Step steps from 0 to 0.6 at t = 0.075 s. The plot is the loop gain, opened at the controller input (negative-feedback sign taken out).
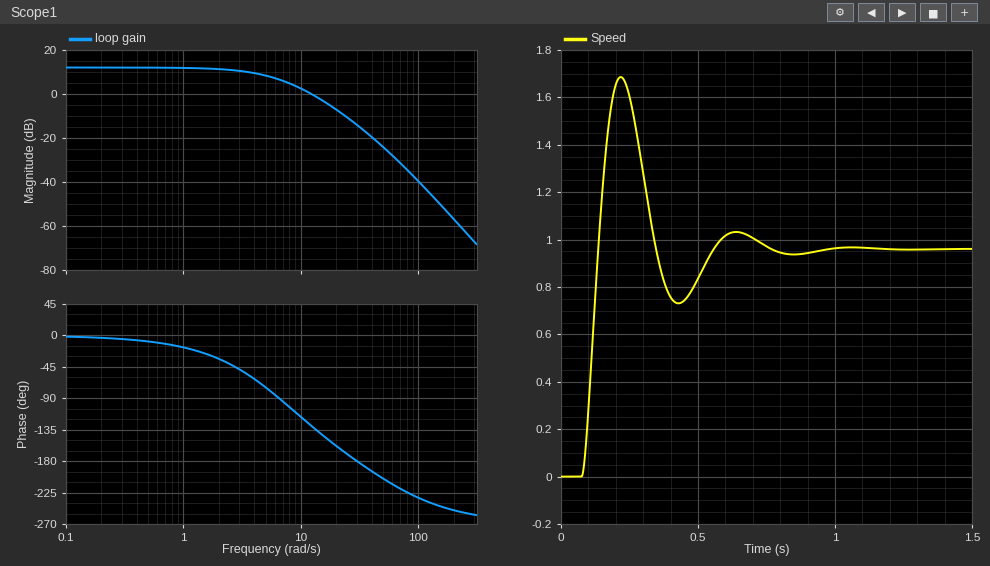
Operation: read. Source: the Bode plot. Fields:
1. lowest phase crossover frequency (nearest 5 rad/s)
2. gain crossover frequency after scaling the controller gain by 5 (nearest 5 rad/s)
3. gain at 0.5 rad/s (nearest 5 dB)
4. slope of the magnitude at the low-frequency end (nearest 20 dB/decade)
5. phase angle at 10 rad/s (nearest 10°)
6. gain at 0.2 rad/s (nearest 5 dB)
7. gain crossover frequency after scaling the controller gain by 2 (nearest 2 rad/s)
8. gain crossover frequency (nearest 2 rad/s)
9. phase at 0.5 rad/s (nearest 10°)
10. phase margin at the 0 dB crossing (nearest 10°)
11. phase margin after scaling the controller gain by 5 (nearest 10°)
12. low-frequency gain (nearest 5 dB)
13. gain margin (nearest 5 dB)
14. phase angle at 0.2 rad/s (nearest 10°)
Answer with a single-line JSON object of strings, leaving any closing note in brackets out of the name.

{"lowest phase crossover frequency": "30 rad/s", "gain crossover frequency after scaling the controller gain by 5": "30 rad/s", "gain at 0.5 rad/s": "10 dB", "slope of the magnitude at the low-frequency end": "0 dB/decade", "phase angle at 10 rad/s": "-120°", "gain at 0.2 rad/s": "10 dB", "gain crossover frequency after scaling the controller gain by 2": "18 rad/s", "gain crossover frequency": "12 rad/s", "phase at 0.5 rad/s": "-10°", "phase margin at the 0 dB crossing": "50°", "phase margin after scaling the controller gain by 5": "0°", "low-frequency gain": "10 dB", "gain margin": "15 dB", "phase angle at 0.2 rad/s": "0°"}
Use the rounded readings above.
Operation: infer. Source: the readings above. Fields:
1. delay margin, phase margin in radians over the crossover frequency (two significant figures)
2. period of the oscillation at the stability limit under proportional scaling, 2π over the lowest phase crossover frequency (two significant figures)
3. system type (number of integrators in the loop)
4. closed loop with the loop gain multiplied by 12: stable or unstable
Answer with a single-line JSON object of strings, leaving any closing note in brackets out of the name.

{"delay margin, phase margin in radians over the crossover frequency": "0.073 s", "period of the oscillation at the stability limit under proportional scaling, 2π over the lowest phase crossover frequency": "0.21 s", "system type": "0", "closed loop with the loop gain multiplied by 12: stable or unstable": "unstable"}
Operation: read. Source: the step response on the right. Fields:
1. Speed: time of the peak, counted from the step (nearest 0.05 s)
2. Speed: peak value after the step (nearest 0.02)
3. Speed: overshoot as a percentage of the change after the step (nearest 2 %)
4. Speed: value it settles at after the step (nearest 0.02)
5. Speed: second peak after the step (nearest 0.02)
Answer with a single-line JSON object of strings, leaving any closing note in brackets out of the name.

{"Speed: time of the peak, counted from the step": "0.15 s", "Speed: peak value after the step": "1.68", "Speed: overshoot as a percentage of the change after the step": "76 %", "Speed: value it settles at after the step": "0.96", "Speed: second peak after the step": "1.04"}
